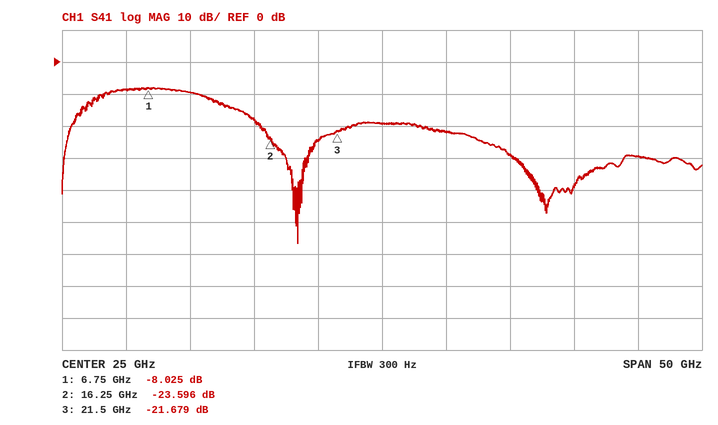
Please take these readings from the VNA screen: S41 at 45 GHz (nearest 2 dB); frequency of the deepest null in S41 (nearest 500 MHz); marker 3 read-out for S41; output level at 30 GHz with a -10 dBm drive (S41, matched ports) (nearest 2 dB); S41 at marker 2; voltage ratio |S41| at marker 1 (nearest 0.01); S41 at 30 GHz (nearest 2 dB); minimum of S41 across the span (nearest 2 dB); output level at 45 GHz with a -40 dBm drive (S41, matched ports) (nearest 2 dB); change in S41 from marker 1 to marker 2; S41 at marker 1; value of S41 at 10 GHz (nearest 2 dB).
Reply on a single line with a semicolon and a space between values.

-30 dB; 18.5 GHz; -21.679 dB; -32 dBm; -23.596 dB; 0.40; -22 dB; -56 dB; -70 dBm; -15.571 dB; -8.025 dB; -10 dB
